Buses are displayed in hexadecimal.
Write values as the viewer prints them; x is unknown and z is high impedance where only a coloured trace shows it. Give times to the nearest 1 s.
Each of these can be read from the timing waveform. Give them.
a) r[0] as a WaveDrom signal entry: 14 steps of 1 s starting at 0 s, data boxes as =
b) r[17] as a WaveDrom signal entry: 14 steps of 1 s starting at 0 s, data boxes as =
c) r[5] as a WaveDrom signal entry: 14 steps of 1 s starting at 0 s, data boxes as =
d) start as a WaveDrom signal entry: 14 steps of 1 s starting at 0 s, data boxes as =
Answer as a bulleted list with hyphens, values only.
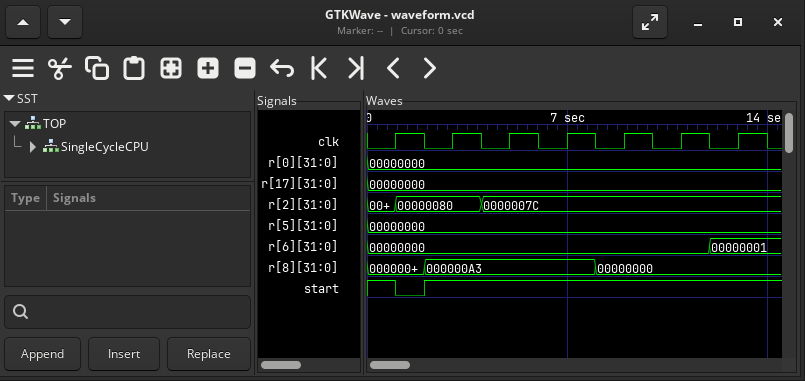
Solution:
- {name: 'r[0]', wave: '=.............', data: '00000000'}
- {name: 'r[17]', wave: '=.............', data: '00000000'}
- {name: 'r[5]', wave: '=.............', data: '00000000'}
- {name: 'start', wave: '101...........'}
